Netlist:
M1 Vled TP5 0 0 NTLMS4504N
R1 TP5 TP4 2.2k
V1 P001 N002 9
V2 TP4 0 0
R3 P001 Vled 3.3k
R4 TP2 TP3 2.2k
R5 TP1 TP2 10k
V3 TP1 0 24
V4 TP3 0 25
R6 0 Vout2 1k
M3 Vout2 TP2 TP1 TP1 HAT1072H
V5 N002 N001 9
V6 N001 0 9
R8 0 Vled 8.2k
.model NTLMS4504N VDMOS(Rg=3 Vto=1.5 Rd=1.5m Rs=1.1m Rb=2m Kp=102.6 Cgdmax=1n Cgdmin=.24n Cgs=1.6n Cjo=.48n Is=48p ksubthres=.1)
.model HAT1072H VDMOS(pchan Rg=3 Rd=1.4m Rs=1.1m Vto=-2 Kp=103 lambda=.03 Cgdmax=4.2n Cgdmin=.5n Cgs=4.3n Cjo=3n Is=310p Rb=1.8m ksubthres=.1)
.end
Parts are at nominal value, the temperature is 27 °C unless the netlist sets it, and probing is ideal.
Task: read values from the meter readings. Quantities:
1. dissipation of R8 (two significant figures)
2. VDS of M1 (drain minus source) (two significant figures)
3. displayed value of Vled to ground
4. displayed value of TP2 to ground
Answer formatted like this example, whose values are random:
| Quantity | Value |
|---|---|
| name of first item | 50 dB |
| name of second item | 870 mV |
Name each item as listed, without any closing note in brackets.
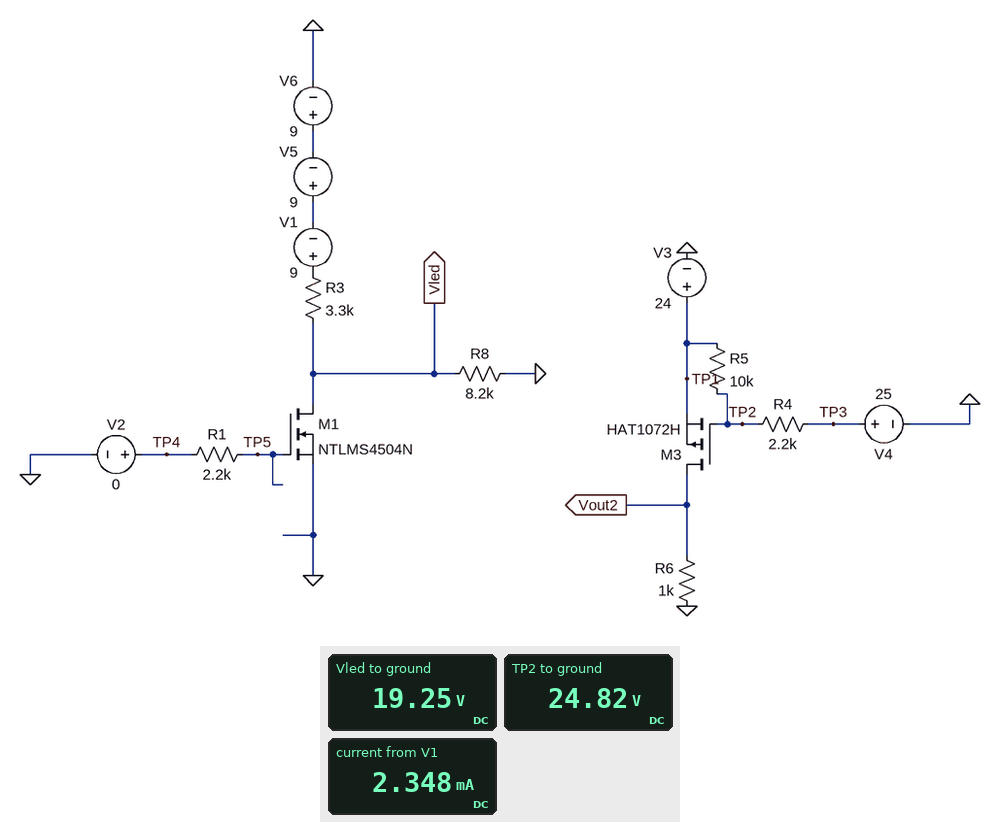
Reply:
| Quantity | Value |
|---|---|
| dissipation of R8 | 45 mW |
| VDS of M1 (drain minus source) | 19 V |
| displayed value of Vled to ground | 19.25 V |
| displayed value of TP2 to ground | 24.82 V |
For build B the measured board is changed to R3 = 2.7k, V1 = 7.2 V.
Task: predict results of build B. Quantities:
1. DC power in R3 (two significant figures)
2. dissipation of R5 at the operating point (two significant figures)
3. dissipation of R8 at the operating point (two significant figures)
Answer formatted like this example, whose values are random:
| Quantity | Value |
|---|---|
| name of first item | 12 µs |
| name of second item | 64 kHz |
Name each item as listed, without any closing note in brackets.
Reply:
| Quantity | Value |
|---|---|
| DC power in R3 | 14 mW |
| dissipation of R5 at the operating point | 67 µW |
| dissipation of R8 at the operating point | 44 mW |
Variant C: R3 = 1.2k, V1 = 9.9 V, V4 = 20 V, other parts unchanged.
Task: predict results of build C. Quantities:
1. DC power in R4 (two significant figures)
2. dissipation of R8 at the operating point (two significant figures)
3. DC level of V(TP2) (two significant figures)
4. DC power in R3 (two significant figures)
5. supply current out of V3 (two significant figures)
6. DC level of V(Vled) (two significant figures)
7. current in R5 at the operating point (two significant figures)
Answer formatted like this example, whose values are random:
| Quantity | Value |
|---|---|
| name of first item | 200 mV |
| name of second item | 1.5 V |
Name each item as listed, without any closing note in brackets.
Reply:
| Quantity | Value |
|---|---|
| DC power in R4 | 240 µW |
| dissipation of R8 at the operating point | 72 mW |
| DC level of V(TP2) | 21 V |
| DC power in R3 | 11 mW |
| supply current out of V3 | 24 mA |
| DC level of V(Vled) | 24 V |
| current in R5 at the operating point | 330 µA |
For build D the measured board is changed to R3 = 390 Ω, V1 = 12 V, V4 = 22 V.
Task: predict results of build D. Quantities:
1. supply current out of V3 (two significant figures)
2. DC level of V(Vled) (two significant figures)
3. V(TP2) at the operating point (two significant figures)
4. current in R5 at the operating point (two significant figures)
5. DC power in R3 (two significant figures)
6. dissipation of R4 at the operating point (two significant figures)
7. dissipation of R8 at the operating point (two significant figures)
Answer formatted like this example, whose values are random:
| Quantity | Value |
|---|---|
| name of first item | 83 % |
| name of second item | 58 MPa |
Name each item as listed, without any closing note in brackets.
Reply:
| Quantity | Value |
|---|---|
| supply current out of V3 | 790 µA |
| DC level of V(Vled) | 29 V |
| V(TP2) at the operating point | 22 V |
| current in R5 at the operating point | 160 µA |
| DC power in R3 | 4.8 mW |
| dissipation of R4 at the operating point | 59 µW |
| dissipation of R8 at the operating point | 100 mW |
